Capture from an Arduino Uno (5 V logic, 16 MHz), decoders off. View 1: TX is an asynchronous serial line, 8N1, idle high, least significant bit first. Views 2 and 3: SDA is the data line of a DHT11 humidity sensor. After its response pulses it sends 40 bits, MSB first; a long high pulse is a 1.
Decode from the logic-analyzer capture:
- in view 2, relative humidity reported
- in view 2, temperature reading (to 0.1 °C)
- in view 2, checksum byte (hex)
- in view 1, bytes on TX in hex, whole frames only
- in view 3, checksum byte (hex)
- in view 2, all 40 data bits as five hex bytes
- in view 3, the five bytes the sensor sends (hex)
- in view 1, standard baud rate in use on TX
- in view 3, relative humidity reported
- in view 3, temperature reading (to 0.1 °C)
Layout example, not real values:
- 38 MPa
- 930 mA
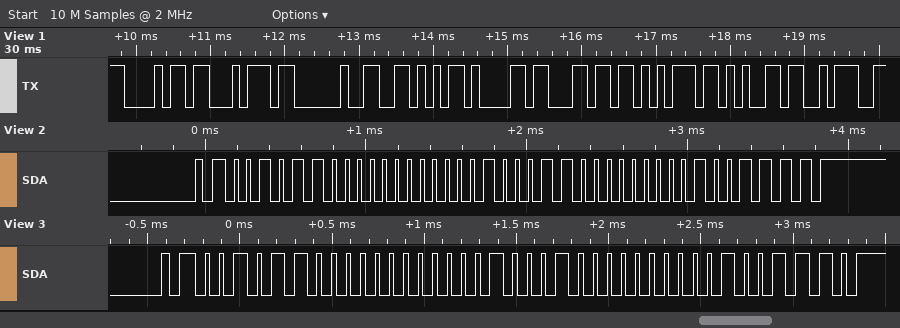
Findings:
- 44 %
- 35.0 °C
- 0x4F
- 0x68 0x74 0x20 0x56 0x61 0x6C 0x75 0x65 0x3A
- 0x4E
- 2C 00 23 00 4F
- 2C 00 22 00 4E
- 9600 baud
- 44 %
- 34.0 °C
